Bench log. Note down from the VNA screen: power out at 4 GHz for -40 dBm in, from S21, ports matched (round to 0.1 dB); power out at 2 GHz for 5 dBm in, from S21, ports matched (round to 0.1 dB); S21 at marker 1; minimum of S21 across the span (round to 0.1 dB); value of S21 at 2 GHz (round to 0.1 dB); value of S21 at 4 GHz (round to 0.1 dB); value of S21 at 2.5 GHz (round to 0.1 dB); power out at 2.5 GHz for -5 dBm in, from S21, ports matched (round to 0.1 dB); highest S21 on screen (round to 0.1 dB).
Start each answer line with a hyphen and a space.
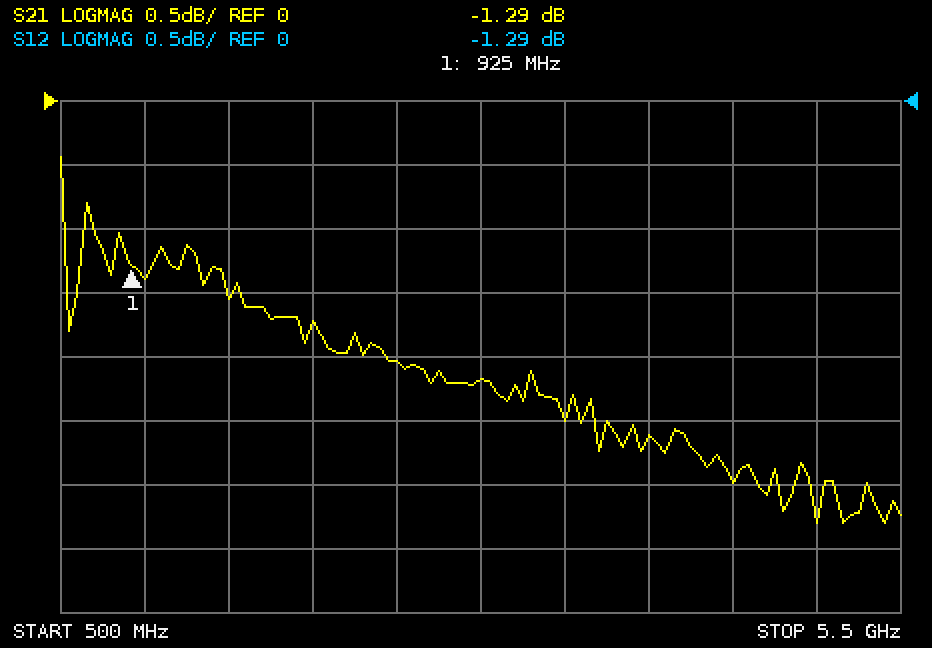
- -42.6 dBm
- 3.3 dBm
- -1.29 dB
- -3.3 dB
- -1.7 dB
- -2.6 dB
- -2.0 dB
- -7.0 dBm
- -0.4 dB
